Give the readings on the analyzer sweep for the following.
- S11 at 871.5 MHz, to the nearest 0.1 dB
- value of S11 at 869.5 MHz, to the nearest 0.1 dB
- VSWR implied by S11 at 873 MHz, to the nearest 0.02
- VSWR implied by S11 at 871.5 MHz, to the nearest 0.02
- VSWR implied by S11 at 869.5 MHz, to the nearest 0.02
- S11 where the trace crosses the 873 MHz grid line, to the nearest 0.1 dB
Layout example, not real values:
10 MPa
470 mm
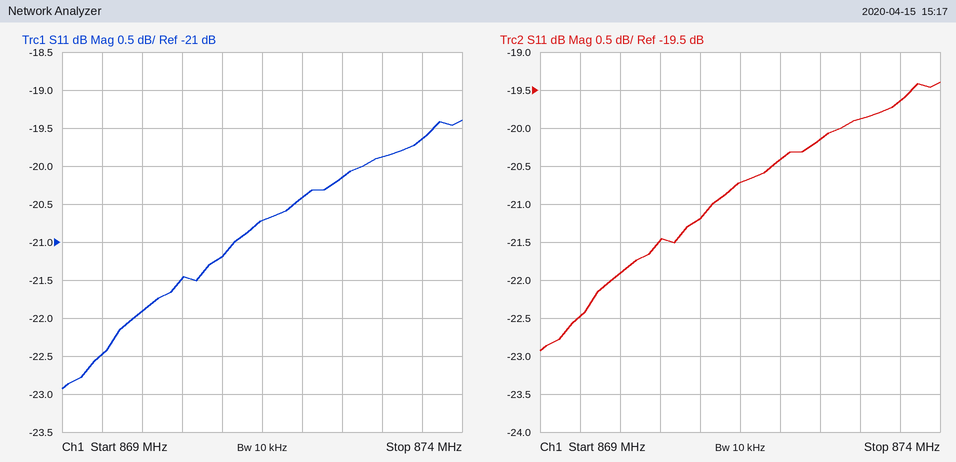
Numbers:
-20.7 dB
-22.5 dB
1.22
1.20
1.16
-19.9 dB
